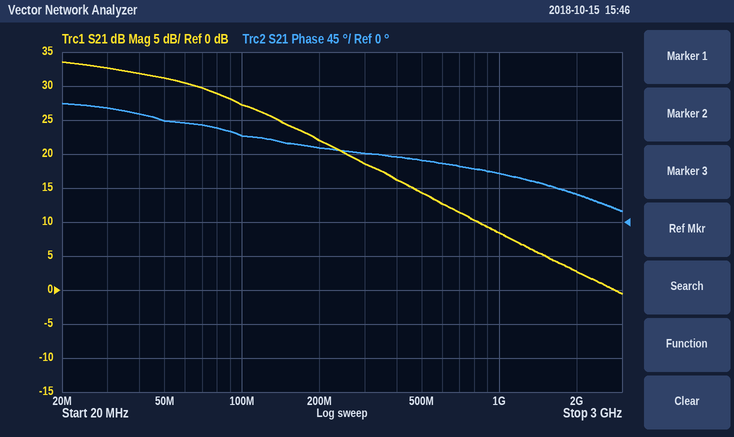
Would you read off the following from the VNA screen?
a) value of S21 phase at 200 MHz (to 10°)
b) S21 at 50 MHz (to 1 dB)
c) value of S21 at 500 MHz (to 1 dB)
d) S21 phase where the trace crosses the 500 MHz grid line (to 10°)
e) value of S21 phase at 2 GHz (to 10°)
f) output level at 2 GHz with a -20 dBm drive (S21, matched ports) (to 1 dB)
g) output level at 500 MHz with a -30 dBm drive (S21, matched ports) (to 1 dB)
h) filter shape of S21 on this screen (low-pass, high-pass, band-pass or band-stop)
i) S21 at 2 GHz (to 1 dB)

100°
31 dB
14 dB
80°
40°
-17 dBm
-16 dBm
low-pass
3 dB
